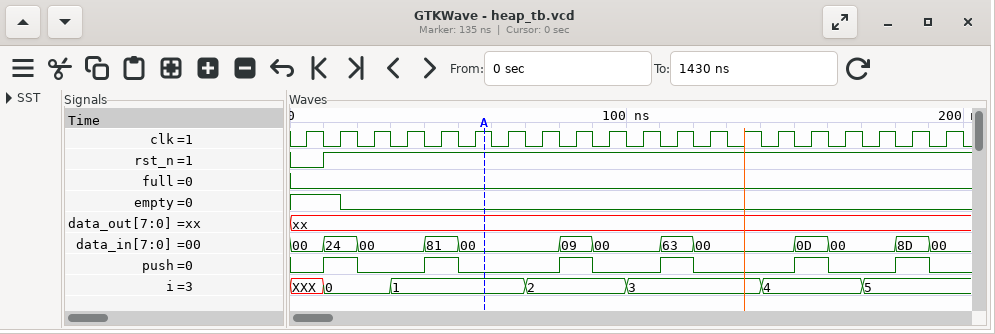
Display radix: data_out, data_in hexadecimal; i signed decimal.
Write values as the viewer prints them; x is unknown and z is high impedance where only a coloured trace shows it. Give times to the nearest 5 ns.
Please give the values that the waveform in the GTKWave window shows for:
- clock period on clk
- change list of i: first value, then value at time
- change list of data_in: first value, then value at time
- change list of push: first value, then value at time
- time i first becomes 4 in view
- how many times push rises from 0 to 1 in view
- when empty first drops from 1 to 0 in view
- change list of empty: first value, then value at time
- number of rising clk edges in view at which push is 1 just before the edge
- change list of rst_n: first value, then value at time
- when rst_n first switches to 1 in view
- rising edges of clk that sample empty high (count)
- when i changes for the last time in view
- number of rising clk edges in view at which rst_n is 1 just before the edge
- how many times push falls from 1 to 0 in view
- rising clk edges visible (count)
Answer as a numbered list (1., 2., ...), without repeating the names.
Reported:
1. 10 ns
2. XXX, 0 at 10 ns, 1 at 30 ns, 2 at 70 ns, 3 at 100 ns, 4 at 140 ns, 5 at 170 ns
3. 00, 24 at 10 ns, 00 at 20 ns, 81 at 40 ns, 00 at 50 ns, 09 at 80 ns, 00 at 90 ns, 63 at 110 ns, 00 at 120 ns, 0D at 150 ns, 00 at 160 ns, 8D at 180 ns, 00 at 190 ns
4. 0, 1 at 10 ns, 0 at 20 ns, 1 at 40 ns, 0 at 50 ns, 1 at 80 ns, 0 at 90 ns, 1 at 110 ns, 0 at 120 ns, 1 at 150 ns, 0 at 160 ns, 1 at 180 ns, 0 at 190 ns
5. 140 ns
6. 6
7. 15 ns
8. 1, 0 at 15 ns
9. 6
10. 0, 1 at 10 ns
11. 10 ns
12. 2
13. 170 ns
14. 19
15. 6
16. 20
